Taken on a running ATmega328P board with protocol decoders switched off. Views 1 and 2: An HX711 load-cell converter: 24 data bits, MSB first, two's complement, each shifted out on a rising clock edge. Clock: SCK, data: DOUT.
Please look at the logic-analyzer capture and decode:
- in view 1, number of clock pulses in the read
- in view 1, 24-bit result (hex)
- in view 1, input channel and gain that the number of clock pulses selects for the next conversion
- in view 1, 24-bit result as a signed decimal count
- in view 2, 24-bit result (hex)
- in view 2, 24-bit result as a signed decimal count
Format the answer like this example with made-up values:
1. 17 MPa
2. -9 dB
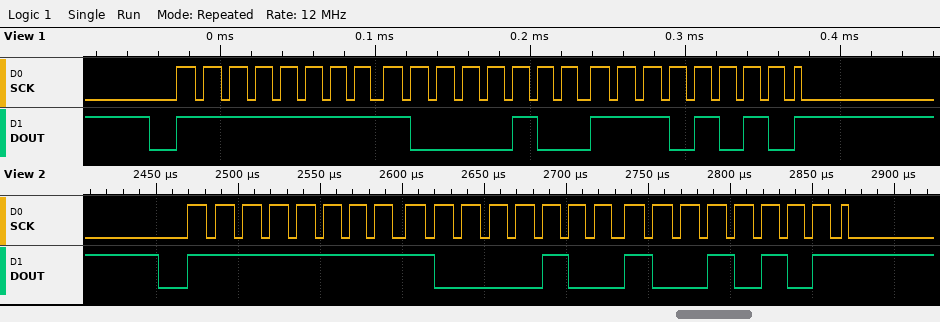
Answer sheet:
1. 25
2. 0xFF84EA
3. channel A, gain 128
4. -31510
5. 0xFF8495
6. -31595
